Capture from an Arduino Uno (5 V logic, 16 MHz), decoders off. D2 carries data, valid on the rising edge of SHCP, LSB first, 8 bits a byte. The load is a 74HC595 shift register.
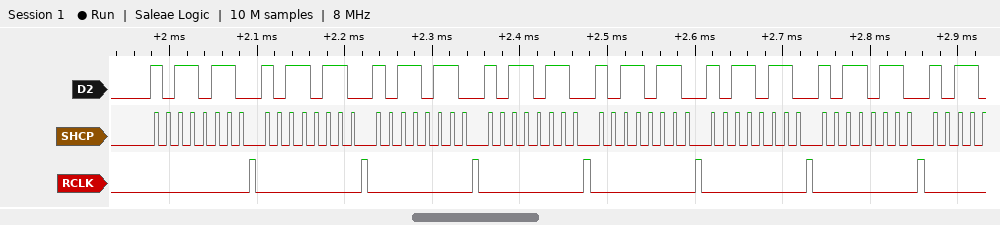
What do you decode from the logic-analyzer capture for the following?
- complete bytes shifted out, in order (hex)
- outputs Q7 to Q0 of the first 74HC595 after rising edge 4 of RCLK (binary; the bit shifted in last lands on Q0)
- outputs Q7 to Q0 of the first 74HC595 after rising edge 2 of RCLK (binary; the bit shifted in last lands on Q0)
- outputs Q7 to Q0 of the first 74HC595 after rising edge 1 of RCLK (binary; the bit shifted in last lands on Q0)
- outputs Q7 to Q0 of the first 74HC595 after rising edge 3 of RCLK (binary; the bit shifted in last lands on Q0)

0x6D 0x6D 0x6D 0x6D 0x6D 0x6D 0x6D
10110110
10110110
10110110
10110110
